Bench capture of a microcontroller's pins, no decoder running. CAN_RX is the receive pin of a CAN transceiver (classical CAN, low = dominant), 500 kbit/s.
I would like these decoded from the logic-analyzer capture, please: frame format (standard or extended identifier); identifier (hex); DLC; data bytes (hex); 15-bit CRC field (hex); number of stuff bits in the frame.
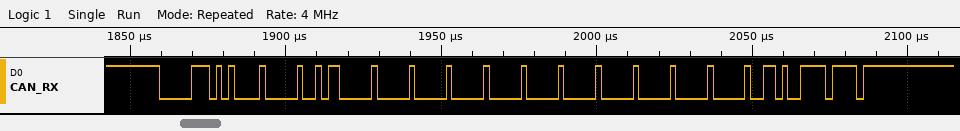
standard
0x06A
8
0B 00 00 00 00 00 00 00
0x34F7
13
